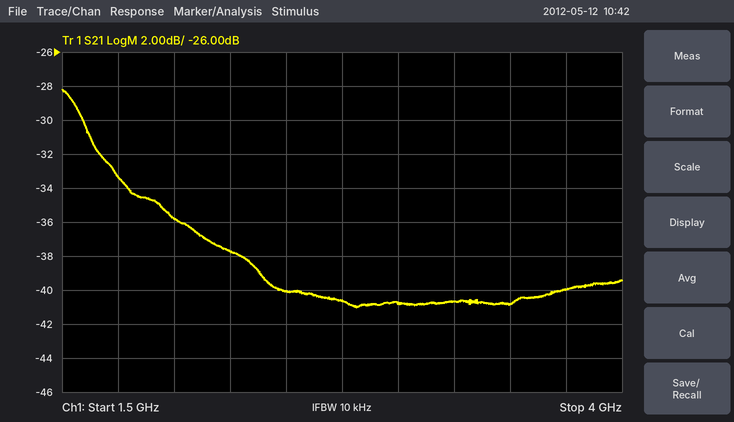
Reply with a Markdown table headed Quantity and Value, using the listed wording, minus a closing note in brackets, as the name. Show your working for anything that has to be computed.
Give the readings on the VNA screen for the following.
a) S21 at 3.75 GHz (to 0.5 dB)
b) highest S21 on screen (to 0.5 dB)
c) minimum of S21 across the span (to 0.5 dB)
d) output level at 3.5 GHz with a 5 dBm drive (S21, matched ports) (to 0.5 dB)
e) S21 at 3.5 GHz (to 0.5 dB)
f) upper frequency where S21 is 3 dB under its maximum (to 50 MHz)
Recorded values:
| Quantity | Value |
|---|---|
| S21 at 3.75 GHz | -40.0 dB |
| highest S21 on screen | -28.0 dB |
| minimum of S21 across the span | -41.0 dB |
| output level at 3.5 GHz with a 5 dBm drive (S21, matched ports) | 5 dBm + (-41.0 dB) = -36.0 dBm |
| S21 at 3.5 GHz | -41.0 dB |
| upper frequency where S21 is 3 dB under its maximum | 1.65 GHz |
